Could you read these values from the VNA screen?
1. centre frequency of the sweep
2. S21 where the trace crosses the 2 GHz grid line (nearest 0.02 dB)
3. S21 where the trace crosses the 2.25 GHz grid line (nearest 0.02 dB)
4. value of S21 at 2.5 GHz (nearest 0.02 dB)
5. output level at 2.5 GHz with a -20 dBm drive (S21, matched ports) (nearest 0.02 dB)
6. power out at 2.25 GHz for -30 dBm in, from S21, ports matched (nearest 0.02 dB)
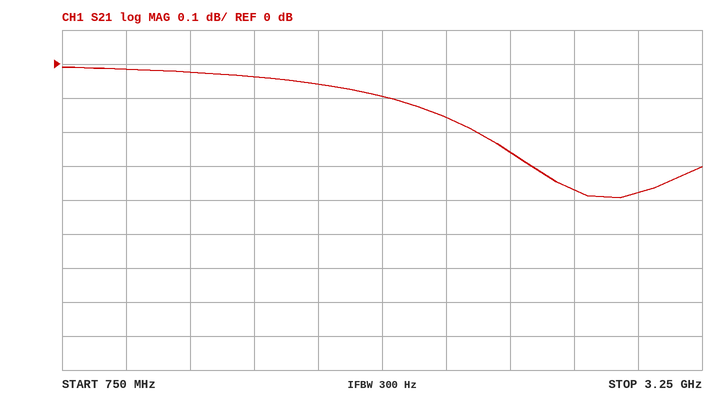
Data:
2 GHz
-0.10 dB
-0.16 dB
-0.26 dB
-20.26 dBm
-30.16 dBm
